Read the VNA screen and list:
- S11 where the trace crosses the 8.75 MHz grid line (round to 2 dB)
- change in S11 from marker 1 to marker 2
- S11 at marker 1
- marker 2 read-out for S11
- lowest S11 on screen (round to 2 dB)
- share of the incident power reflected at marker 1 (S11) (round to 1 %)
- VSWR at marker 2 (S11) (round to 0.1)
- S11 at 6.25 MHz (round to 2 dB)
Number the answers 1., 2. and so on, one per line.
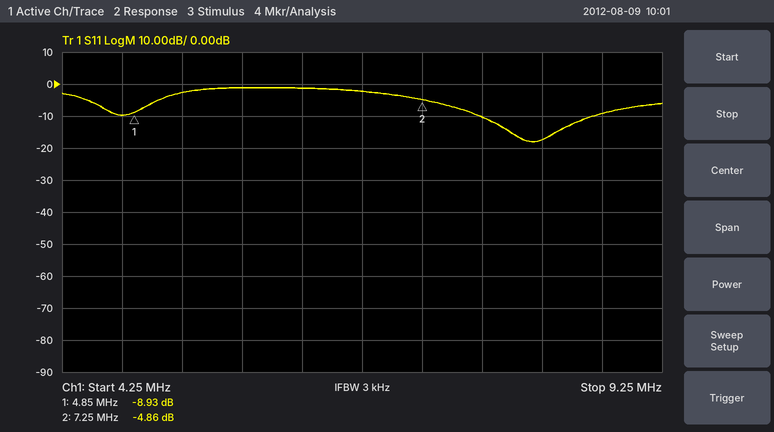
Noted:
1. -10 dB
2. 4.07 dB
3. -8.93 dB
4. -4.86 dB
5. -18 dB
6. 13 %
7. 3.7
8. -2 dB
